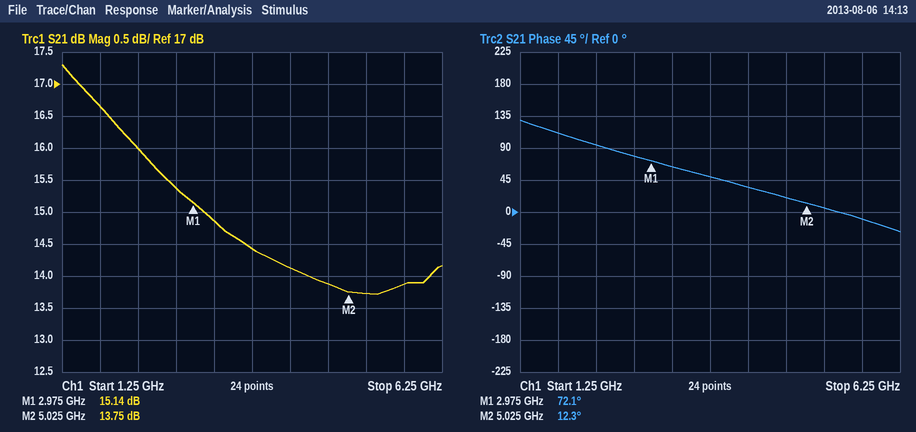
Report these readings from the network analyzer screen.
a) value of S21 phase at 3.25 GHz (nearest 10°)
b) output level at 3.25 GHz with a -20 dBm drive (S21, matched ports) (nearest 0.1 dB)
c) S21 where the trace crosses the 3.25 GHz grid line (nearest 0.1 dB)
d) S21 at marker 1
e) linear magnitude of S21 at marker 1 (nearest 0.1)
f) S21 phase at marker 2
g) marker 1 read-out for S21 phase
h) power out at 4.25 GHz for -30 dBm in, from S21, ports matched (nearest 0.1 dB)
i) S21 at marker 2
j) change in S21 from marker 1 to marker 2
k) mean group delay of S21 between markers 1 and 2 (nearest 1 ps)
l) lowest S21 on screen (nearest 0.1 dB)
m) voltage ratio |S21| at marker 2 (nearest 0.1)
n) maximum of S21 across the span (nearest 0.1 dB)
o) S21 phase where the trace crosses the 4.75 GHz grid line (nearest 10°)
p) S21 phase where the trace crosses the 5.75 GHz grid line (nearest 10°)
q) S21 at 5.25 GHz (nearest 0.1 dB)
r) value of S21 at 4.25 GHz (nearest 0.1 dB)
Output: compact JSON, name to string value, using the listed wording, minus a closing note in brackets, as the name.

{"value of S21 phase at 3.25 GHz": "60°", "output level at 3.25 GHz with a -20 dBm drive (S21, matched ports)": "-5.1 dBm", "S21 where the trace crosses the 3.25 GHz grid line": "14.9 dB", "S21 at marker 1": "15.14 dB", "linear magnitude of S21 at marker 1": "5.7", "S21 phase at marker 2": "12.3°", "marker 1 read-out for S21 phase": "72.1°", "power out at 4.25 GHz for -30 dBm in, from S21, ports matched": "-15.9 dBm", "S21 at marker 2": "13.75 dB", "change in S21 from marker 1 to marker 2": "-1.39 dB", "mean group delay of S21 between markers 1 and 2": "81 ps", "lowest S21 on screen": "13.7 dB", "voltage ratio |S21| at marker 2": "4.9", "maximum of S21 across the span": "17.3 dB", "S21 phase where the trace crosses the 4.75 GHz grid line": "20°", "S21 phase where the trace crosses the 5.75 GHz grid line": "-10°", "S21 at 5.25 GHz": "13.7 dB", "value of S21 at 4.25 GHz": "14.1 dB"}
